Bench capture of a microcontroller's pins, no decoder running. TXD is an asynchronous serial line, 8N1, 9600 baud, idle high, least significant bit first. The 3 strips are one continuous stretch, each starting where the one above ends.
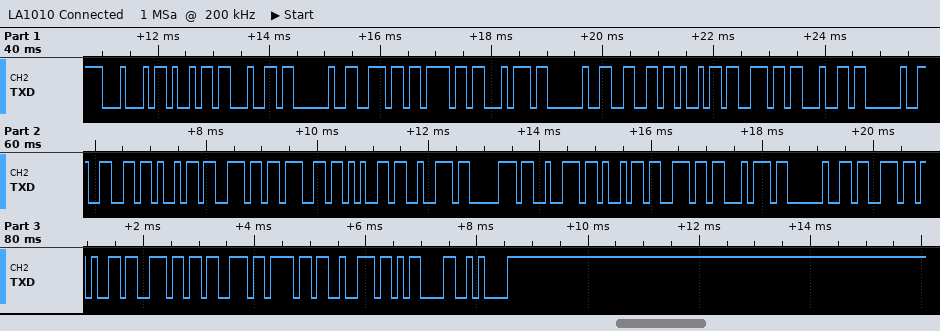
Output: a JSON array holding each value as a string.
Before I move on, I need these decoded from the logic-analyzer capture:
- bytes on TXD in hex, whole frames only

["44 69 64 20 6E 6F 74 20 66 69 6E 64 20 66 69 6E 67 65 72 70 72 69 6E 74 20 73 65 6E 73 6F 72 0D 0A"]
